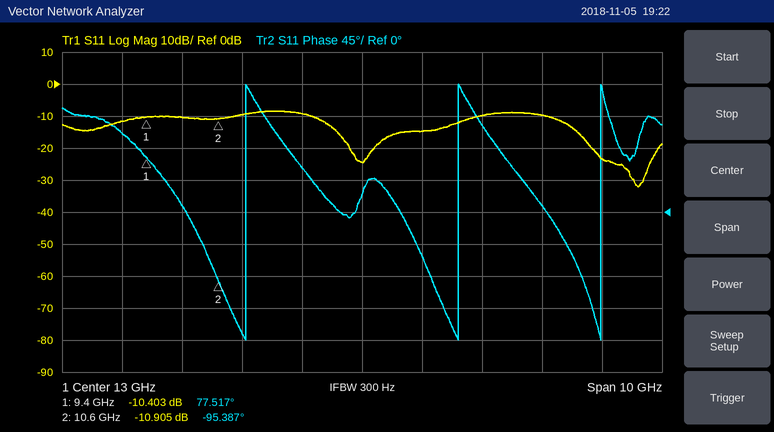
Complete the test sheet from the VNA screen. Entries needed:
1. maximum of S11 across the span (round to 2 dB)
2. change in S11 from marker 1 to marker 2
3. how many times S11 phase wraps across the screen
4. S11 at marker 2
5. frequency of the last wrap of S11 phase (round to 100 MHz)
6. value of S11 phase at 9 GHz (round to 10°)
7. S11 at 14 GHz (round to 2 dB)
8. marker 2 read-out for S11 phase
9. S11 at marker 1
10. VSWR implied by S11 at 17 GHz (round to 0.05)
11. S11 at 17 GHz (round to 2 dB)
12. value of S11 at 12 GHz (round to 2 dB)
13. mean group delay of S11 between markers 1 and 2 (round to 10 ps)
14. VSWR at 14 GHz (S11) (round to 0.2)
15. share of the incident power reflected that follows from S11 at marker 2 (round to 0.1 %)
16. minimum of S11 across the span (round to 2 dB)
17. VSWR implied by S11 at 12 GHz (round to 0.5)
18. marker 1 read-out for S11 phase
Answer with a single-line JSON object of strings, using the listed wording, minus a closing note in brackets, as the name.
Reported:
{"maximum of S11 across the span": "-8 dB", "change in S11 from marker 1 to marker 2": "-0.502 dB", "how many times S11 phase wraps across the screen": "3", "S11 at marker 2": "-10.905 dB", "frequency of the last wrap of S11 phase": "17.0 GHz", "value of S11 phase at 9 GHz": "110°", "S11 at 14 GHz": "-14 dB", "marker 2 read-out for S11 phase": "-95.387°", "S11 at marker 1": "-10.403 dB", "VSWR implied by S11 at 17 GHz": "1.15", "S11 at 17 GHz": "-24 dB", "value of S11 at 12 GHz": "-10 dB", "mean group delay of S11 between markers 1 and 2": "400 ps", "VSWR at 14 GHz (S11)": "1.4", "share of the incident power reflected that follows from S11 at marker 2": "8.1 %", "minimum of S11 across the span": "-32 dB", "VSWR implied by S11 at 12 GHz": "2.0", "marker 1 read-out for S11 phase": "77.517°"}
